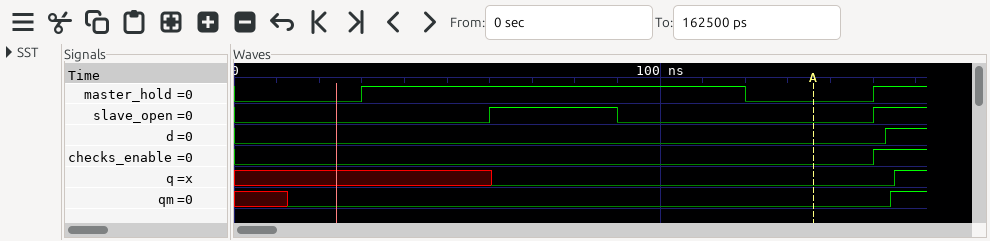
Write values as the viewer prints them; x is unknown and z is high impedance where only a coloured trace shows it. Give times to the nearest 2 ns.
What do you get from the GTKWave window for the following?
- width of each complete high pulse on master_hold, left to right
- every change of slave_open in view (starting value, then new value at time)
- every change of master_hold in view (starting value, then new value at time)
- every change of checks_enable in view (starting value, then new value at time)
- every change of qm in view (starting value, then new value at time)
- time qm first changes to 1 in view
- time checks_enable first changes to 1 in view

90 ns
0, 1 at 60 ns, 0 at 90 ns, 1 at 150 ns
0, 1 at 30 ns, 0 at 120 ns, 1 at 150 ns
0, 1 at 150 ns
x, 0 at 12 ns, 1 at 154 ns
154 ns
150 ns
